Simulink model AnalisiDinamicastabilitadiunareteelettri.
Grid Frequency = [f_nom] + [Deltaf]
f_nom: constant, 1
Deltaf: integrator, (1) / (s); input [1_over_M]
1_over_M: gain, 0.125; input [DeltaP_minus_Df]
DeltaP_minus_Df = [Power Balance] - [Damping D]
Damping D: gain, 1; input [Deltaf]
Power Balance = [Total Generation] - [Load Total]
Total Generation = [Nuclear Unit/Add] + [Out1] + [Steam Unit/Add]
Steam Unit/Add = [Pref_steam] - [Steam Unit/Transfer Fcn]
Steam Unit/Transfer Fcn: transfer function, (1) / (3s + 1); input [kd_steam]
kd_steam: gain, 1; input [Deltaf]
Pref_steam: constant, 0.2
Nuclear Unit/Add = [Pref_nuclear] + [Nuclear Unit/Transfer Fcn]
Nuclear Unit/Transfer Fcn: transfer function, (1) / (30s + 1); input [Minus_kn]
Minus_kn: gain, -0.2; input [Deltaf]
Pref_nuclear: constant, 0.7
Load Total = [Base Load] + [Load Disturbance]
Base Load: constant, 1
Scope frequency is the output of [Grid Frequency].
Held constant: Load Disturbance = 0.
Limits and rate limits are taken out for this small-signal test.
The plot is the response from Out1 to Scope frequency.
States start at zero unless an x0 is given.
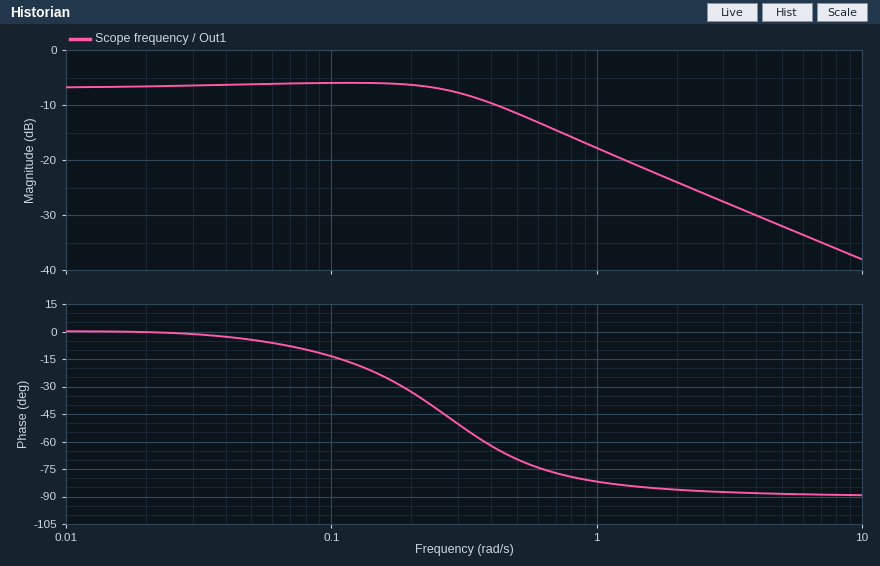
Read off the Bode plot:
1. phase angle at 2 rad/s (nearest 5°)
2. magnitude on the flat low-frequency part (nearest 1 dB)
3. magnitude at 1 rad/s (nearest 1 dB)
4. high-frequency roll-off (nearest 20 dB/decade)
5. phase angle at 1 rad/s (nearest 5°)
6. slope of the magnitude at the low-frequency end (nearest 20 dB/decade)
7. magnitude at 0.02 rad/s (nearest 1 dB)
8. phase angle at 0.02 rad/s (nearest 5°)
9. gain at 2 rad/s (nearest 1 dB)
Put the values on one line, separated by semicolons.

-85°; -7 dB; -18 dB; -20 dB/decade; -80°; 0 dB/decade; -7 dB; 0°; -24 dB
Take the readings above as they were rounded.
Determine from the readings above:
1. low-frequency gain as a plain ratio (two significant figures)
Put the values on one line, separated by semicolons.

0.45
